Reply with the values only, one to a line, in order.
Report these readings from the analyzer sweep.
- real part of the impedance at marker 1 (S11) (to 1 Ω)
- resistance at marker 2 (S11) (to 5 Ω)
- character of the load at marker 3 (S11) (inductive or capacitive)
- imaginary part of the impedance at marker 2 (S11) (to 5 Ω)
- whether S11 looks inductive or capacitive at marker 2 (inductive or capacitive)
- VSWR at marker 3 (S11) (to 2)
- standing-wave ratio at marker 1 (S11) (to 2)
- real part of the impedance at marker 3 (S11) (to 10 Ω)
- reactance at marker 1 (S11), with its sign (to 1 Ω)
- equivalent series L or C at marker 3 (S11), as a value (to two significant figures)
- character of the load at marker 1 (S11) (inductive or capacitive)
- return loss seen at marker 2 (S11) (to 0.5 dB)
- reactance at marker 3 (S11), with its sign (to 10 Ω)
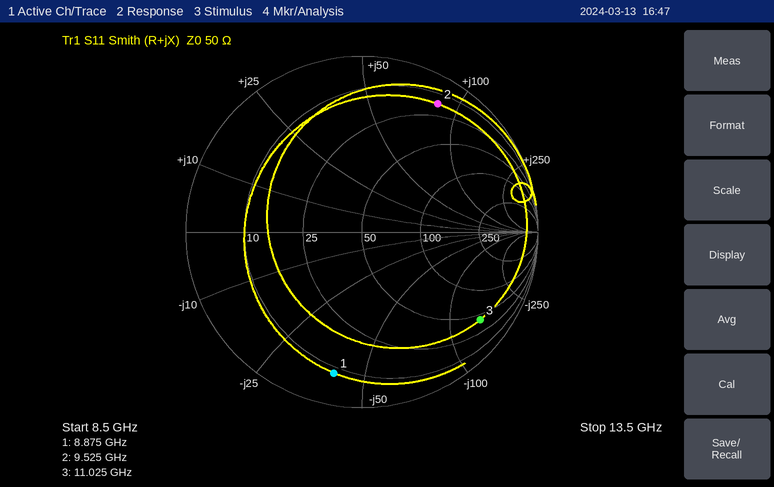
8 Ω
15 Ω
capacitive
+85 Ω
inductive
12
10
40 Ω
-40 Ω
100 fF
capacitive
1.5 dB
-140 Ω
